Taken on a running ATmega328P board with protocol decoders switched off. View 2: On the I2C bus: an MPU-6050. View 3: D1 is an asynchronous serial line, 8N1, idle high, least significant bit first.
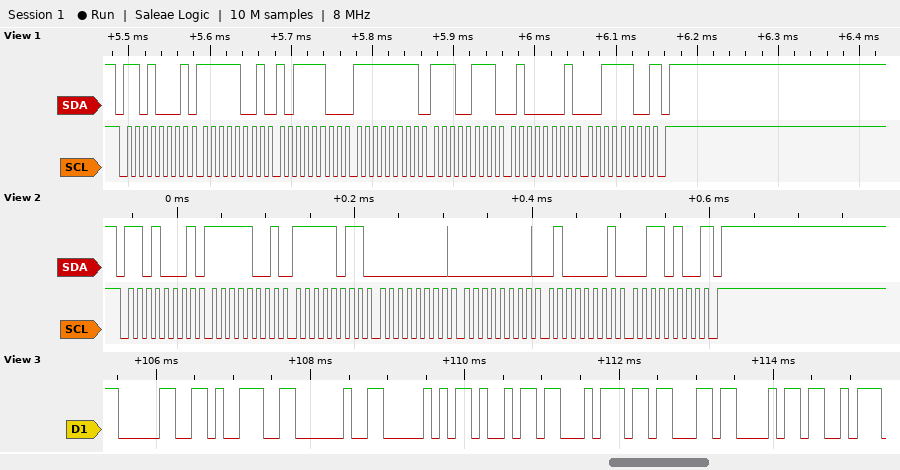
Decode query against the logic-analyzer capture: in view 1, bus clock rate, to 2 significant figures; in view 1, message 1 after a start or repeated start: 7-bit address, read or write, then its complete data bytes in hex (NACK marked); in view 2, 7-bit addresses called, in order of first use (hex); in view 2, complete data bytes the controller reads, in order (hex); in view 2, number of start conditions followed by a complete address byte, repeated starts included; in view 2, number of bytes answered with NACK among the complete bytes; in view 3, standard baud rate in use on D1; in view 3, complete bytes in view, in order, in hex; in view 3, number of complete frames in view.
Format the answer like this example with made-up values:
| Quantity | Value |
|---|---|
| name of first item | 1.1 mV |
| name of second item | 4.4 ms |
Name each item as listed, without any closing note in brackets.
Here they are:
| Quantity | Value |
|---|---|
| in view 1, bus clock rate, to 2 significant figures | 100 kHz |
| in view 1, message 1 after a start or repeated start: 7-bit address, read or write, then its complete data bytes in hex | 0x68 read: F9 BC FF E7 41 3C NACK |
| in view 2, 7-bit addresses called, in order of first use | 0x68 |
| in view 2, complete data bytes the controller reads, in order | F9 FB 00 00 41 34 |
| in view 2, number of start conditions followed by a complete address byte, repeated starts included | 1 |
| in view 2, number of bytes answered with NACK among the complete bytes | 1 |
| in view 3, standard baud rate in use on D1 | 9600 baud |
| in view 3, complete bytes in view, in order, in hex | 30 39 20 50 69 74 63 68 |
| in view 3, number of complete frames in view | 8 |
